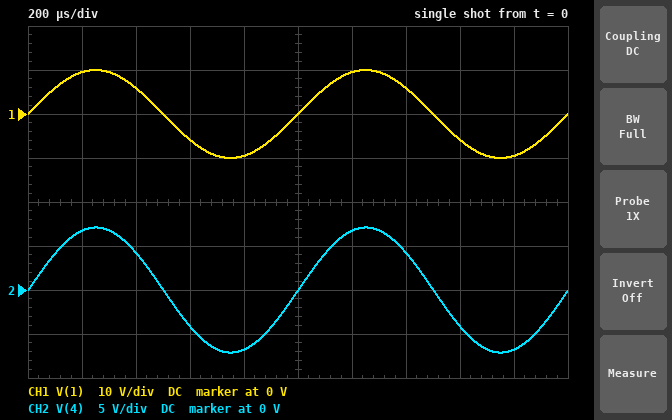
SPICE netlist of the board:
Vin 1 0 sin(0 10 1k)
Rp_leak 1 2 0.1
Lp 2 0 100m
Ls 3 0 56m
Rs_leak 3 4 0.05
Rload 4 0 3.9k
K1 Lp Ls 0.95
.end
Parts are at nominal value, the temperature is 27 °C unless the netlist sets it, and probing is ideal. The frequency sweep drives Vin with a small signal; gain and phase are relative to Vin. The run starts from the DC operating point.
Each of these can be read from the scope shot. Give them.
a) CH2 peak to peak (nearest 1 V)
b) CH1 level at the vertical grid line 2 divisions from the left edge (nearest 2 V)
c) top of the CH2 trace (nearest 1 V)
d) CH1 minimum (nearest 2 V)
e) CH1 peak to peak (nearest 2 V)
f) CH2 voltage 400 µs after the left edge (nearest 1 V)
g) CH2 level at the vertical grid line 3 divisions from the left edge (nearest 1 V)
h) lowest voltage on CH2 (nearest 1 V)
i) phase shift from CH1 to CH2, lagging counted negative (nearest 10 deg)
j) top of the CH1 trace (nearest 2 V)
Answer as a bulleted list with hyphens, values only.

- 14 V
- 6 V
- 7 V
- -10 V
- 20 V
- 4 V
- -4 V
- -7 V
- 0 deg
- 10 V
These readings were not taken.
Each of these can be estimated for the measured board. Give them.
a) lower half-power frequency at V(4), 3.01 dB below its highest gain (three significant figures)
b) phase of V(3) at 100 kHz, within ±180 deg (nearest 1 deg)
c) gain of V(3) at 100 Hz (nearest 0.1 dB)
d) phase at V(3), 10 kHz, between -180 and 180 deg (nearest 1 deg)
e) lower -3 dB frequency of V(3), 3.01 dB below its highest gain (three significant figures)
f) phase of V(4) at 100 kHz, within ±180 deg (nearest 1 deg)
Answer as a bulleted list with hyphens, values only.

- 159 mHz
- -41 deg
- -3.0 dB
- -5 deg
- 159 mHz
- -41 deg
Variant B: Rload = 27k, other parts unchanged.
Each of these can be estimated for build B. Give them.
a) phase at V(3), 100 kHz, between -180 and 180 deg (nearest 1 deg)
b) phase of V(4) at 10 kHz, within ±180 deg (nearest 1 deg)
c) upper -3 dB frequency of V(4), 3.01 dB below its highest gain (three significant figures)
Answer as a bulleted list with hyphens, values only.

- -7 deg
- -1 deg
- 787 kHz
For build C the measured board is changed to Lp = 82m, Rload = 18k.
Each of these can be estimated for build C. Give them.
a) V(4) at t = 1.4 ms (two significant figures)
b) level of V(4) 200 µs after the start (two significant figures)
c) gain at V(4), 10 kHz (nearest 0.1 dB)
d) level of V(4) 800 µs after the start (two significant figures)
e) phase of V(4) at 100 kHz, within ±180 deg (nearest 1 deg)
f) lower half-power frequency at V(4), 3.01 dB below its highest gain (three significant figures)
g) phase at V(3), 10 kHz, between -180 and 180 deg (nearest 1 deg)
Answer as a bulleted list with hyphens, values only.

- 4.6 V
- 7.5 V
- -2.1 dB
- -7.5 V
- -11 deg
- 194 mHz
- -1 deg
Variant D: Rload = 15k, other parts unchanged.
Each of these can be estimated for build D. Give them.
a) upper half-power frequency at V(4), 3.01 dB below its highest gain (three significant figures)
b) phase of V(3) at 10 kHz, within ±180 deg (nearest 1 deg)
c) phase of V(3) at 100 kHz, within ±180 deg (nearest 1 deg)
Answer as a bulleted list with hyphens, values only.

- 437 kHz
- -1 deg
- -13 deg
